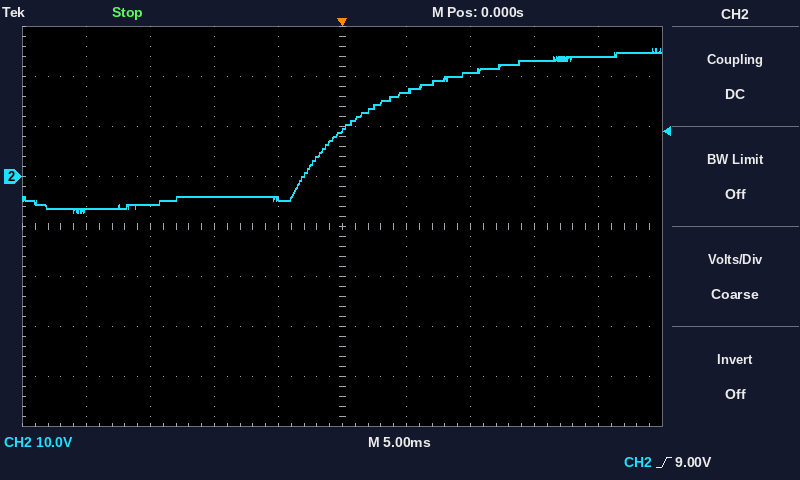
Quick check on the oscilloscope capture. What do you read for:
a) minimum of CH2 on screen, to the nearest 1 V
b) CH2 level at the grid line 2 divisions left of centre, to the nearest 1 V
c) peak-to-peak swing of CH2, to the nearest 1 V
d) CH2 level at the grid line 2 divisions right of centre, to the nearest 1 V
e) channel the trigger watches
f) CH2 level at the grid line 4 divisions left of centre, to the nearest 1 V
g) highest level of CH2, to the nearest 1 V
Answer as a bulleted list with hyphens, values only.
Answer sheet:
- -7 V
- -4 V
- 33 V
- 21 V
- CH2
- -7 V
- 26 V
